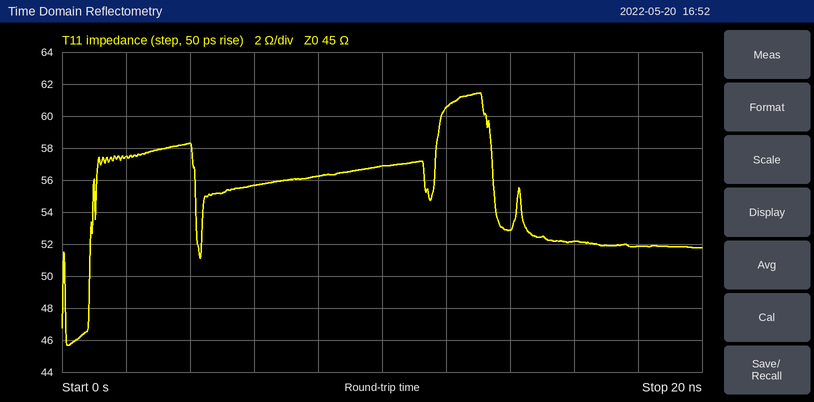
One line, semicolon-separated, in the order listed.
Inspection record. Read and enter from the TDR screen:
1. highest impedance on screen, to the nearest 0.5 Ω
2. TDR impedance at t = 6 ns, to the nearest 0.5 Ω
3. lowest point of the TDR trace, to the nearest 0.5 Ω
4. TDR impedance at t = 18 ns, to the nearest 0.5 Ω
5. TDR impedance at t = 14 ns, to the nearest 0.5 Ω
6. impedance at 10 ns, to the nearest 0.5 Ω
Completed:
61.5 Ω; 55.5 Ω; 45.5 Ω; 52.0 Ω; 53.0 Ω; 57.0 Ω
